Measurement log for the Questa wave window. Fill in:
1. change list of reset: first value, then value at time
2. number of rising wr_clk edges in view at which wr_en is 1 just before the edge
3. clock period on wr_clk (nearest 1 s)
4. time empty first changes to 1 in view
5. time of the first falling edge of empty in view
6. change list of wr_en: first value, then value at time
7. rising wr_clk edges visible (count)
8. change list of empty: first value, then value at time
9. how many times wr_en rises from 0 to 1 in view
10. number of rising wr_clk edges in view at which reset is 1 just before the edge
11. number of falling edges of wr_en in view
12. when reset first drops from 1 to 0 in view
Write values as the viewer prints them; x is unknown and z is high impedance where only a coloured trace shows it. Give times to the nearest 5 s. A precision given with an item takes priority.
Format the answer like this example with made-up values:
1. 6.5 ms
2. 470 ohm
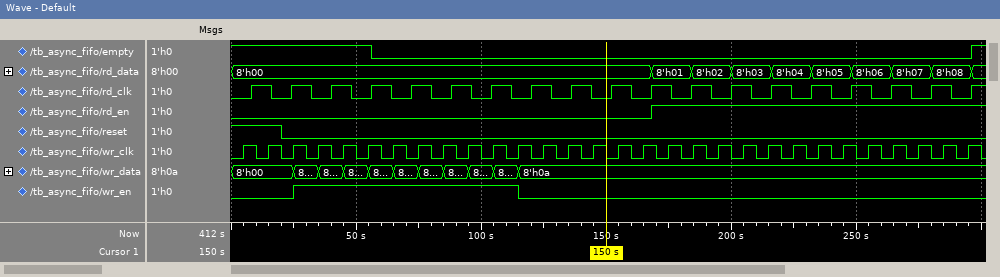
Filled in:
1. 1, 0 at 20 s
2. 9
3. 10 s
4. 295 s
5. 55 s
6. 0, 1 at 25 s, 0 at 115 s
7. 30
8. 1, 0 at 55 s, 1 at 295 s
9. 1
10. 2
11. 1
12. 20 s
